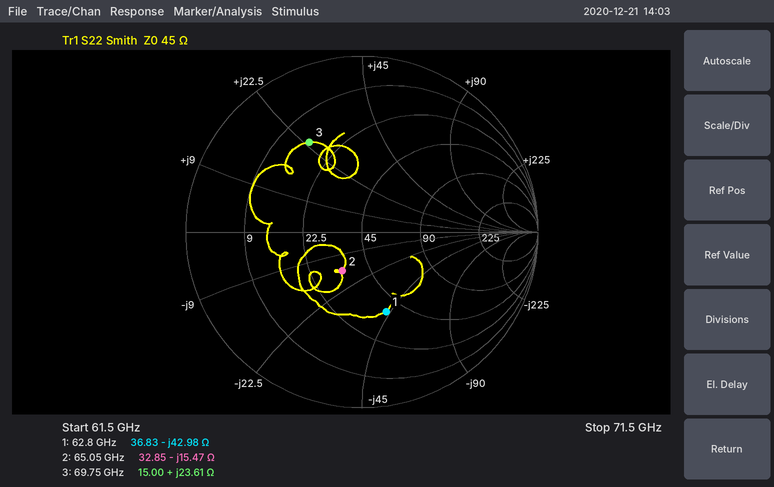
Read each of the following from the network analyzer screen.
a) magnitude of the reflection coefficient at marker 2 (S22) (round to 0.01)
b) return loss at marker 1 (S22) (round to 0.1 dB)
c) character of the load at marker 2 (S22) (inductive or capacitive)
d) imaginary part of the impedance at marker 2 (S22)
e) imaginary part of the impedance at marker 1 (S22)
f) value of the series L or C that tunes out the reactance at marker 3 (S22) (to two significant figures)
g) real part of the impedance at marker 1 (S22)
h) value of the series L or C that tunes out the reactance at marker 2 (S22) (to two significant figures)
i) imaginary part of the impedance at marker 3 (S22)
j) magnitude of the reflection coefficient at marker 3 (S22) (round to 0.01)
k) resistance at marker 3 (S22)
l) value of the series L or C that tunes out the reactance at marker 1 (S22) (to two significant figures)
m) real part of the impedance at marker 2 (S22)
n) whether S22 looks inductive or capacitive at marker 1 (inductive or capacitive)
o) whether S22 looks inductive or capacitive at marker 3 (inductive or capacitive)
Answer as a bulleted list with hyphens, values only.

- 0.25
- 6.5 dB
- capacitive
- -15.47 Ω
- -42.98 Ω
- 97 fF
- 36.83 Ω
- 38 pH
- +23.61 Ω
- 0.59
- 15.00 Ω
- 110 pH
- 32.85 Ω
- capacitive
- inductive
